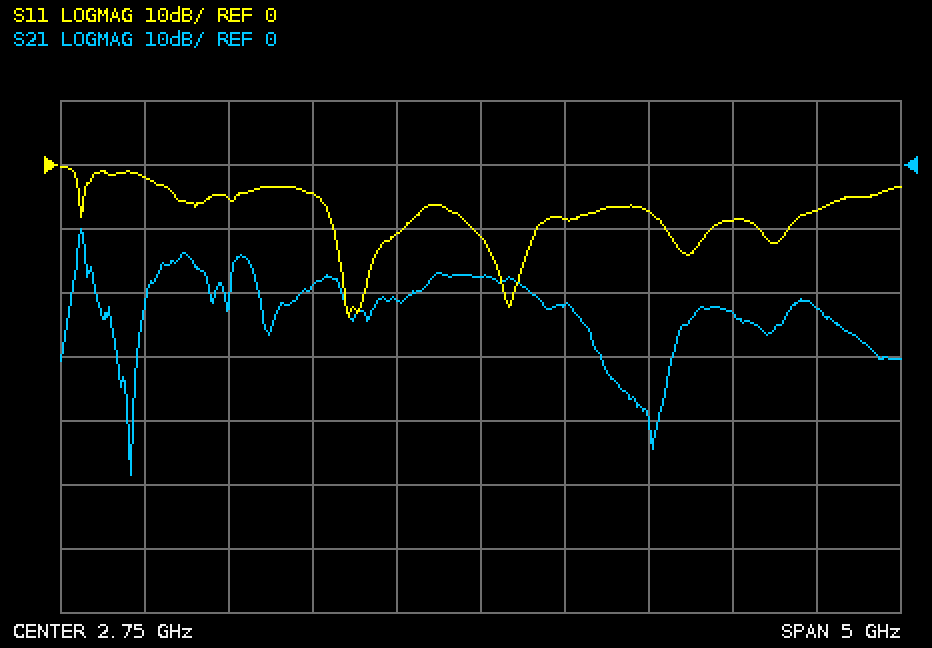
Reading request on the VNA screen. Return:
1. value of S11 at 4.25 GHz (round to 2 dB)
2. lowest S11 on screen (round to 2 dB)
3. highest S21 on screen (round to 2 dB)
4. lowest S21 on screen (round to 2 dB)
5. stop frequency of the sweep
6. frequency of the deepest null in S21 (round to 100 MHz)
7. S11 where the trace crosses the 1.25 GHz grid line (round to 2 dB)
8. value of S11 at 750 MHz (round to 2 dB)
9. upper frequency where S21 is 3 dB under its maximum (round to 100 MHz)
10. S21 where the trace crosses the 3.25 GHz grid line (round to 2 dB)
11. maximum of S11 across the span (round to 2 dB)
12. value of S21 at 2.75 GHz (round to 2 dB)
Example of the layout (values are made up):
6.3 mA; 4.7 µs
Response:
-8 dB; -24 dB; -10 dB; -48 dB; 5.25 GHz; 700 MHz; -6 dB; -2 dB; 400 MHz; -22 dB; 0 dB; -18 dB
